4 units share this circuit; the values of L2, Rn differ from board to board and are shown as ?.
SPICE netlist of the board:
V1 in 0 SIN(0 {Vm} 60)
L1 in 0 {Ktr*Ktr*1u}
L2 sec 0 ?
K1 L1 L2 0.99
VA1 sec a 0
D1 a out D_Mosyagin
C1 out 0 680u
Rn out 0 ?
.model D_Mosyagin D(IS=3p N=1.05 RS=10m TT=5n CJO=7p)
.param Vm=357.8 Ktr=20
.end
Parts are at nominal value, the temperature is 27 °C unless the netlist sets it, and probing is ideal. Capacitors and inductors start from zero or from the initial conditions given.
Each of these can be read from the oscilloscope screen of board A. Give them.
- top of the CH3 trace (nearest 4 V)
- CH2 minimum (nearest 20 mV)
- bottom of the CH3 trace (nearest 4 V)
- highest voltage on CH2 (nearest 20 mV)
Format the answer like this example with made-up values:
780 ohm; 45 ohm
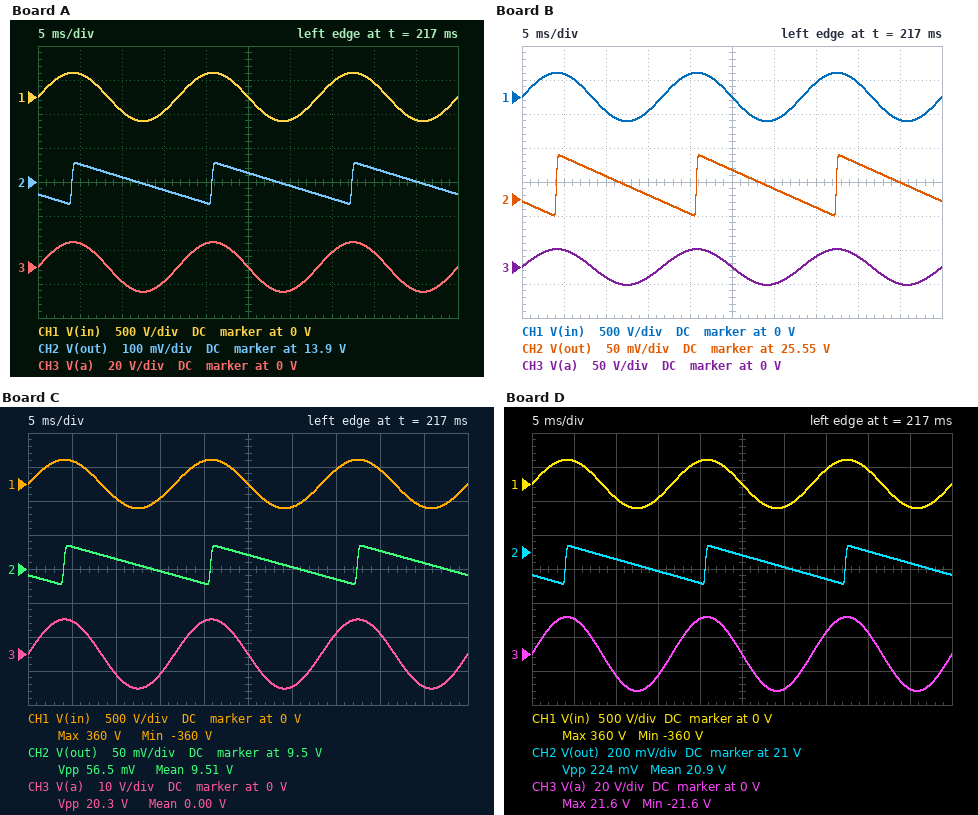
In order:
16 V; 13.84 V; -16 V; 13.96 V
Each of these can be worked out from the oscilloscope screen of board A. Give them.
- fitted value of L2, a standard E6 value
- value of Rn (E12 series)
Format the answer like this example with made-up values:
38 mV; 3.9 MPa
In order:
680 nH; 2.7 kΩ
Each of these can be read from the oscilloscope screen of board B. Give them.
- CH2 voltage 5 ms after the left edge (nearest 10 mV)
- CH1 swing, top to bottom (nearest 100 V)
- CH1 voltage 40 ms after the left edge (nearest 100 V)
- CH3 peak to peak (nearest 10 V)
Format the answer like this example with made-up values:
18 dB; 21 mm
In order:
25.61 V; 700 V; 200 V; 50 V
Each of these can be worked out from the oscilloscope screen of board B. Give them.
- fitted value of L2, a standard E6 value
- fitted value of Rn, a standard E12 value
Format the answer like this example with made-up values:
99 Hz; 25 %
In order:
2.2 µH; 6.8 kΩ
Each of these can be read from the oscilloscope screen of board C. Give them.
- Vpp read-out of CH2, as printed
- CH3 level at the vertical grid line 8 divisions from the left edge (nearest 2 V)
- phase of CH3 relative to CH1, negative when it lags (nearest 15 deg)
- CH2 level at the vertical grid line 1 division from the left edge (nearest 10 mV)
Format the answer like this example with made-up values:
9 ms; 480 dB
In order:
56.5 mV; 6 V; 0 deg; 9.53 V
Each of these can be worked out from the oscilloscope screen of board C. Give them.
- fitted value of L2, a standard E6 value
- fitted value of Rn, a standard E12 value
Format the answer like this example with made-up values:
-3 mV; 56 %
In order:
330 nH; 3.9 kΩ
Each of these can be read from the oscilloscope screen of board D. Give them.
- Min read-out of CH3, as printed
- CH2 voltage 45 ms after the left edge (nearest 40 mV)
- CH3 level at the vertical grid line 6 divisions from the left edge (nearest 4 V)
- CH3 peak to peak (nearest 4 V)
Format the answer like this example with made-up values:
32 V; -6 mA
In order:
-21.6 V; 20.92 V; -20 V; 44 V
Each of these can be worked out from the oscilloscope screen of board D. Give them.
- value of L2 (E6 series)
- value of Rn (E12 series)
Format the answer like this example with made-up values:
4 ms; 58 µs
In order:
1.5 µH; 2.2 kΩ
